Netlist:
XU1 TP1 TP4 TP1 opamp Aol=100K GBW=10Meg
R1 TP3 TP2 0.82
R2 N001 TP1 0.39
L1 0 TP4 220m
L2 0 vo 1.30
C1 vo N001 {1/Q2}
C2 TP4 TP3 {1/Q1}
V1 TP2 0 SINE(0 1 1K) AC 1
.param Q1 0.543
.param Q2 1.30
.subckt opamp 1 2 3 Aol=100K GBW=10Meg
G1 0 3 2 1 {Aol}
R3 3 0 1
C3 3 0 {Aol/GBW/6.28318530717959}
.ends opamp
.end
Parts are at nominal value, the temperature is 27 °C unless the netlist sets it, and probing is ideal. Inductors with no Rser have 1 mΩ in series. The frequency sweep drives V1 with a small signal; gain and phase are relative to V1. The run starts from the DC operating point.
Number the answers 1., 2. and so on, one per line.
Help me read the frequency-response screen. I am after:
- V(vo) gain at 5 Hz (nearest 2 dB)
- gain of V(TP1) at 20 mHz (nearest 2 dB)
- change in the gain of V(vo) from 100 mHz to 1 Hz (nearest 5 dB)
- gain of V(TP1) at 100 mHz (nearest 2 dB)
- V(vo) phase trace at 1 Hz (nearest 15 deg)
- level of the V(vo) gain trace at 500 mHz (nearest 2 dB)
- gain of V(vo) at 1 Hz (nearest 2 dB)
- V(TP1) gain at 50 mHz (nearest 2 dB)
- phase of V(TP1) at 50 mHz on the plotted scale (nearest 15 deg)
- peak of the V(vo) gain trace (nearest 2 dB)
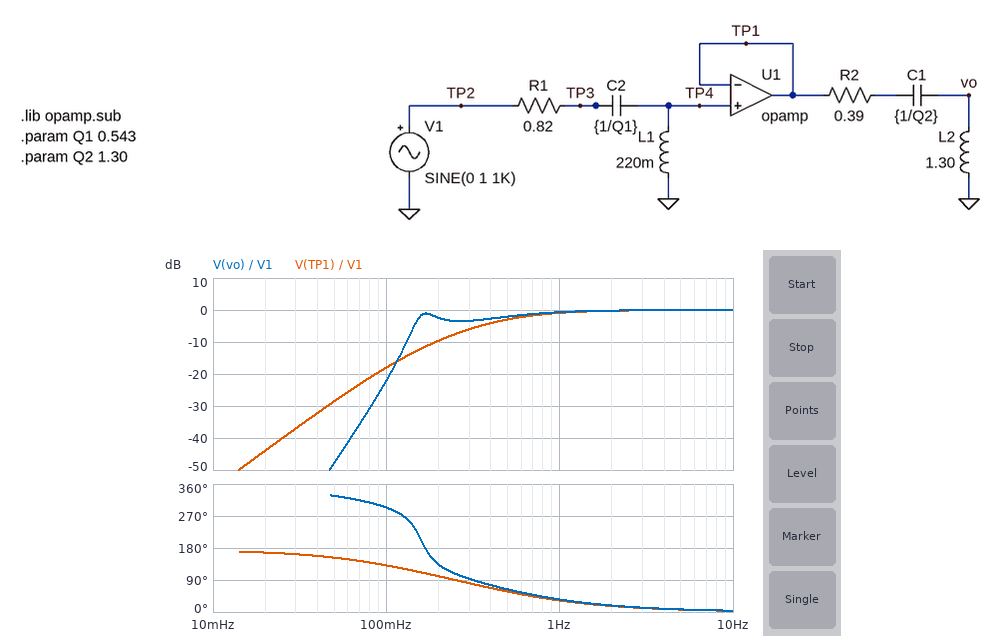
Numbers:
1. 0 dB
2. -44 dB
3. 20 dB
4. -18 dB
5. 30 deg
6. -2 dB
7. 0 dB
8. -28 dB
9. 150 deg
10. 0 dB
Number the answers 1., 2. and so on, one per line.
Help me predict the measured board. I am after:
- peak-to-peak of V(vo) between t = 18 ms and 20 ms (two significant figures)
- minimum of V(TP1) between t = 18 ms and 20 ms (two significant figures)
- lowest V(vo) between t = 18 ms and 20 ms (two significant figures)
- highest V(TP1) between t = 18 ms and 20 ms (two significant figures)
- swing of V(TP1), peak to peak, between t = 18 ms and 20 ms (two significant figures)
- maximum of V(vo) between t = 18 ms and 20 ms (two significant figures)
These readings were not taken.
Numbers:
1. 2.0 V
2. -1.0 V
3. -1.0 V
4. 1.0 V
5. 2.0 V
6. 1.0 V
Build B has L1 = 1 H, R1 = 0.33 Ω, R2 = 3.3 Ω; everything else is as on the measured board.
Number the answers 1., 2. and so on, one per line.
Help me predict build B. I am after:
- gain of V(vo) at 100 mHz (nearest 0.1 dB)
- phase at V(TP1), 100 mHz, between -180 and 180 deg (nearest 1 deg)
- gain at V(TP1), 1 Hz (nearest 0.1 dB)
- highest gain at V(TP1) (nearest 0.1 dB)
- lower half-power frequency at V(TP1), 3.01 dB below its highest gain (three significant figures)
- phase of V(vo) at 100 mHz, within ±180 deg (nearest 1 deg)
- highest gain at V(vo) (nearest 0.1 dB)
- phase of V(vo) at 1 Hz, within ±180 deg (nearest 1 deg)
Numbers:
1. -8.9 dB
2. 125 deg
3. 0.1 dB
4. 7.2 dB
5. 101 mHz
6. -124 deg
7. 0 dB
8. 26 deg
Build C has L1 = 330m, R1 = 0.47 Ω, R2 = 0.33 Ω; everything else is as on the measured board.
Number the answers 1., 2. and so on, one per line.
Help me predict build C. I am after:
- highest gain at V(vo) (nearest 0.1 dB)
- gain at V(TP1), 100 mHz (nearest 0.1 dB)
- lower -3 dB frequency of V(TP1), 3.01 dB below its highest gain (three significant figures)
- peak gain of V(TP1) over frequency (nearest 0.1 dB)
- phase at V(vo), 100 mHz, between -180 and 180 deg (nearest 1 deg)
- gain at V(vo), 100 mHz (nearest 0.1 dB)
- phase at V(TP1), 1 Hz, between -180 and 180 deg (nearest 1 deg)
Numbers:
1. 8.5 dB
2. -11.8 dB
3. 179 mHz
4. 0.7 dB
5. -51 deg
6. -15.8 dB
7. 13 deg
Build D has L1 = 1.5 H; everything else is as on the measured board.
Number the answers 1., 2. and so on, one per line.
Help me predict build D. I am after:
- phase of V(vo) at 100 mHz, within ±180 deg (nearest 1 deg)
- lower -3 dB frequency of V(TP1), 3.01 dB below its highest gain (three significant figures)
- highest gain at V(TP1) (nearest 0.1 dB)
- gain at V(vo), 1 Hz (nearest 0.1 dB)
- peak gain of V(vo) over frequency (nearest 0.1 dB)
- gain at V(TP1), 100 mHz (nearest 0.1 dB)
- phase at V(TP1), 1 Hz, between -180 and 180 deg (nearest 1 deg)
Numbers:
1. -113 deg
2. 81.0 mHz
3. 1.8 dB
4. 0.3 dB
5. 12.0 dB
6. 1.2 dB
7. 5 deg
